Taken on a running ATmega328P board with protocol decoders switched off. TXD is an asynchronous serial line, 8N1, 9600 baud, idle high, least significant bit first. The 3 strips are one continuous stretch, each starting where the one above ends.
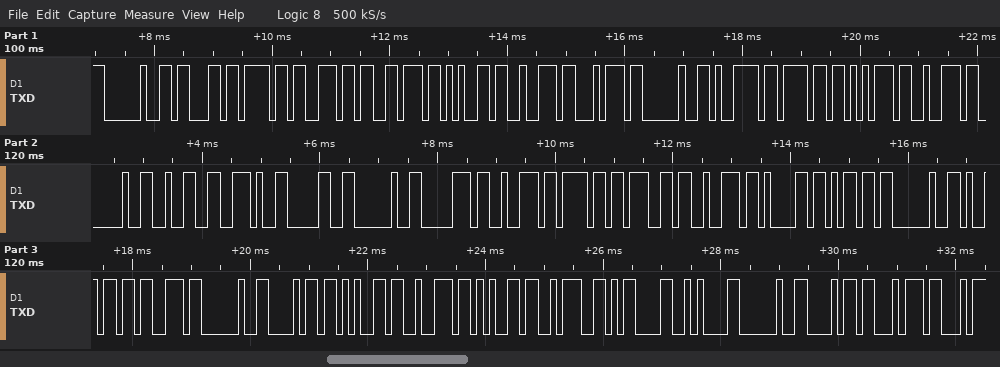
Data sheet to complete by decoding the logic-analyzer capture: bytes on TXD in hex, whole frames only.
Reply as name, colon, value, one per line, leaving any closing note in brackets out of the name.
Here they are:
bytes on TXD in hex, whole frames only: 20 63 6F 6E 76 65 72 74 20 79 6F 75 72 20 32 2E 30 20 70 72 6F 67 72 61 6D 20 69 73 20 68 65 72 65 3A 0D 0A 20 68 74
